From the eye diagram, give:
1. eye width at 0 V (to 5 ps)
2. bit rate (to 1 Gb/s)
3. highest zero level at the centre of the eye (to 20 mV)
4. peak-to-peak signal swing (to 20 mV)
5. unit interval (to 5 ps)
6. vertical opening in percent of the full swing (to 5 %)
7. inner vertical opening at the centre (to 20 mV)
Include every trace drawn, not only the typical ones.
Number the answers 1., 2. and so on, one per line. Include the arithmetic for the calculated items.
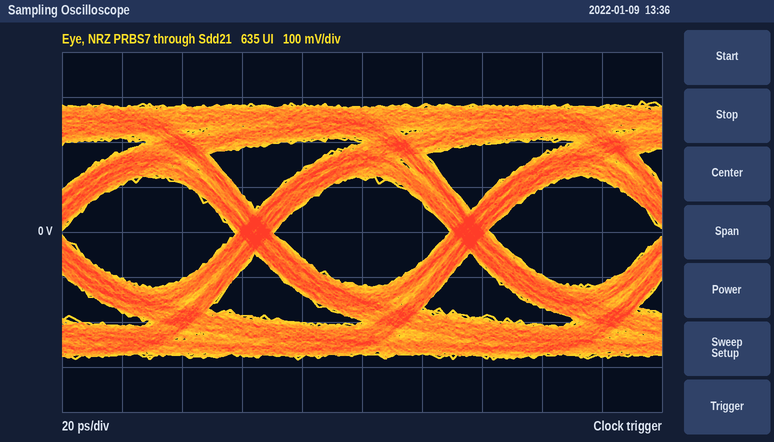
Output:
1. 60 ps
2. 14 Gb/s
3. -120 mV
4. 580 mV
5. 70 ps
6. 240 mV / 580 mV ≈ 41.4 %, so 40 % to the nearest 5 %
7. 240 mV
